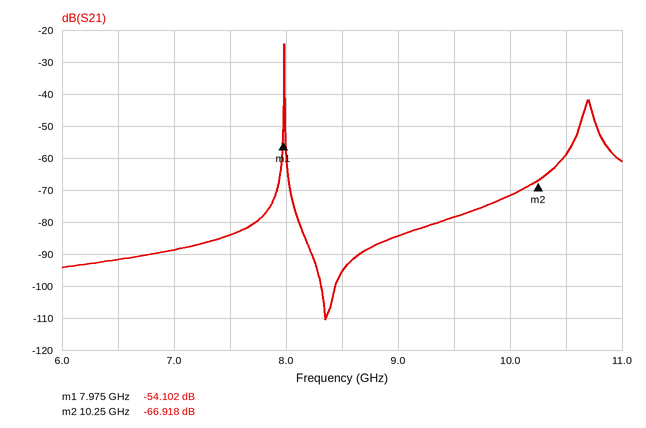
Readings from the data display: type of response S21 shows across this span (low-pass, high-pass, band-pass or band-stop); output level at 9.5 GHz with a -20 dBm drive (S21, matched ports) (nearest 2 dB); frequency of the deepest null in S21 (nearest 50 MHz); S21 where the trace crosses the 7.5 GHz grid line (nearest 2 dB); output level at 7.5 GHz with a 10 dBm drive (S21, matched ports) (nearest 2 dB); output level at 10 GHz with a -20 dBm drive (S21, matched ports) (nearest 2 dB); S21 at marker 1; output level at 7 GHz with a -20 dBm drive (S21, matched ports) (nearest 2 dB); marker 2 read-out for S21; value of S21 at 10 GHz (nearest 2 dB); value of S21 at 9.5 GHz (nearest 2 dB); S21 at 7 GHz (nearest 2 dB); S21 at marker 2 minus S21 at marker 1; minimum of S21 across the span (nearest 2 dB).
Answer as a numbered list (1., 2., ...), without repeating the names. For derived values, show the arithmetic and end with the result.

1. band-pass
2. -20 dBm + (-78 dB) = -98 dBm
3. 8.35 GHz
4. -84 dB
5. 10 dBm + (-84 dB) = -74 dBm
6. -20 dBm + (-72 dB) = -92 dBm
7. -54.102 dB
8. -20 dBm + (-88 dB) = -108 dBm
9. -66.918 dB
10. -72 dB
11. -78 dB
12. -88 dB
13. -66.918 − (-54.102) = -12.816 dB
14. -110 dB
